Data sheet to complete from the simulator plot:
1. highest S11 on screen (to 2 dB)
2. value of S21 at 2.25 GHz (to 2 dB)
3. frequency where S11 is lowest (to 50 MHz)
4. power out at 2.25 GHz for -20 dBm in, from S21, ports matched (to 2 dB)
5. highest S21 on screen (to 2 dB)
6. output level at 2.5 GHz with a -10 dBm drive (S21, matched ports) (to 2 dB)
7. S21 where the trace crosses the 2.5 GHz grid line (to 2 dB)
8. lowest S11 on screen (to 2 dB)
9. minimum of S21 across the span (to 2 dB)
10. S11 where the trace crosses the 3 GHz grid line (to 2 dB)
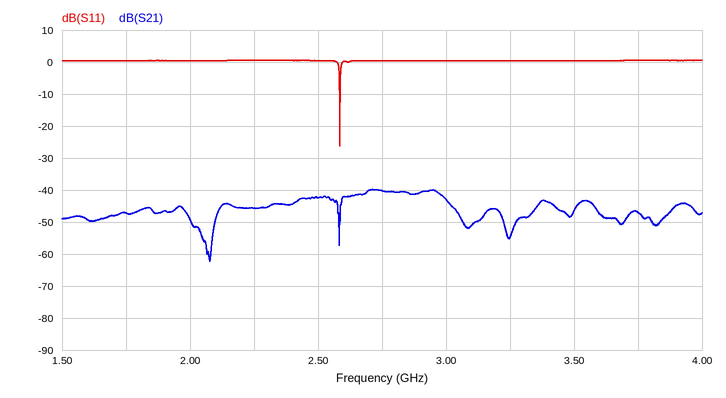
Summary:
0 dB
-46 dB
2.60 GHz
-66 dBm
-40 dB
-52 dBm
-42 dB
-26 dB
-62 dB
0 dB
